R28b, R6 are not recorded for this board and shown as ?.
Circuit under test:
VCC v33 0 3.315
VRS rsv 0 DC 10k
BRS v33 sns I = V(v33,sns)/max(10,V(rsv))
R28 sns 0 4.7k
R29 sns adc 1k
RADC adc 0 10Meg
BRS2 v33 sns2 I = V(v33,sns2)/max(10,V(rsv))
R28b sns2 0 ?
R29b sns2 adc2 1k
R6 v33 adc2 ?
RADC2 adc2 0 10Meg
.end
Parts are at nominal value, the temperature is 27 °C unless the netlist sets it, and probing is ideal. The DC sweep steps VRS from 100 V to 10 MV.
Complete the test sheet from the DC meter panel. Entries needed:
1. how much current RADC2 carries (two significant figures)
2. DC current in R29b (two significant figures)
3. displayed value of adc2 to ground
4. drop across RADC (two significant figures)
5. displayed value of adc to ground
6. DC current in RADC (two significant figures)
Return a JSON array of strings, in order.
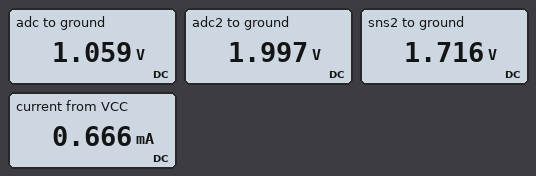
["200 nA", "280 µA", "1.997 V", "1.1 V", "1.059 V", "110 nA"]
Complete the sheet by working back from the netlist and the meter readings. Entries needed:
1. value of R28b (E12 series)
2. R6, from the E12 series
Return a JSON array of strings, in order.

["3.9 kΩ", "4.7 kΩ"]
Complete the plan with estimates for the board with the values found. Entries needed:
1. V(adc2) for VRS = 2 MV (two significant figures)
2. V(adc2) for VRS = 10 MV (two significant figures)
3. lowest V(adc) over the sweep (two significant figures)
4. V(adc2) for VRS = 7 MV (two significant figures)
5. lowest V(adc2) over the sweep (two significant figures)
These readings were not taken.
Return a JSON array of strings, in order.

["1.7 V", "1.7 V", "1.6 mV", "1.7 V", "1.7 V"]
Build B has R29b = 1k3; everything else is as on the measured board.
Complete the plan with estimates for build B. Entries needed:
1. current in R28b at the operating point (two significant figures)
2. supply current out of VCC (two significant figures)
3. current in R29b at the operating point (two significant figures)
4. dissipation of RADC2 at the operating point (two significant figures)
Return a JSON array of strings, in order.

["430 µA", "660 µA", "270 µA", "420 nW"]
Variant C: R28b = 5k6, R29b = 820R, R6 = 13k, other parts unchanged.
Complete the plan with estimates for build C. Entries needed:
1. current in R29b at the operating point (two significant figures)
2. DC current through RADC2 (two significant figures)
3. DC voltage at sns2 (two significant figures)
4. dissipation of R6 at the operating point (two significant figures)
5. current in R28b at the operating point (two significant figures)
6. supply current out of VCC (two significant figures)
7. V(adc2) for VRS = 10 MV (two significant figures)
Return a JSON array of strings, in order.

["120 µA", "170 nA", "1.6 V", "190 µW", "290 µA", "520 µA", "1.1 V"]
